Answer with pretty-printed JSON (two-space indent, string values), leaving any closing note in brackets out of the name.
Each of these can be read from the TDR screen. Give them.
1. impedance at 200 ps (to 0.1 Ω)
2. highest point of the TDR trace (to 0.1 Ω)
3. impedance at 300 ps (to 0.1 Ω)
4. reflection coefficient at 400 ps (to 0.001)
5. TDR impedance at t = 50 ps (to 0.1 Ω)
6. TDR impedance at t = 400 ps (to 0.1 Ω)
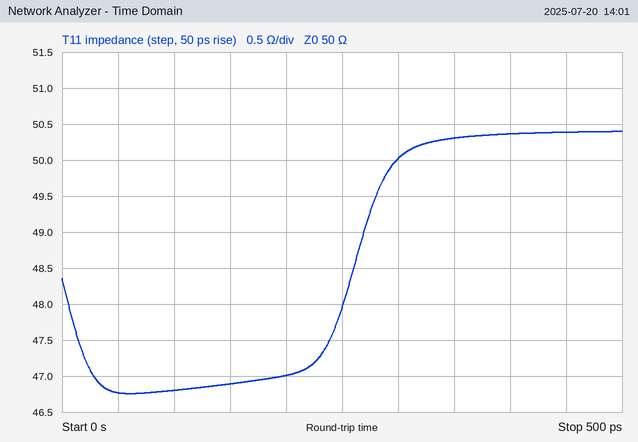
{
  "impedance at 200 ps": "47.0 Ω",
  "highest point of the TDR trace": "50.4 Ω",
  "impedance at 300 ps": "50.0 Ω",
  "reflection coefficient at 400 ps": "+0.004",
  "TDR impedance at t = 50 ps": "46.8 Ω",
  "TDR impedance at t = 400 ps": "50.4 Ω"
}
